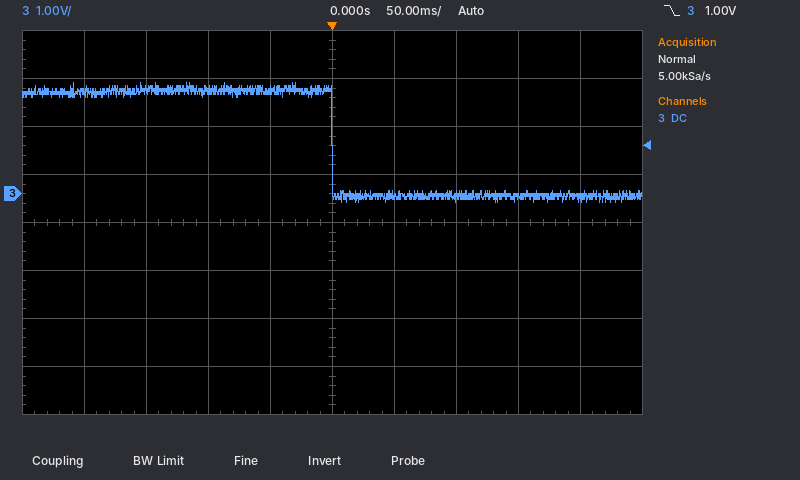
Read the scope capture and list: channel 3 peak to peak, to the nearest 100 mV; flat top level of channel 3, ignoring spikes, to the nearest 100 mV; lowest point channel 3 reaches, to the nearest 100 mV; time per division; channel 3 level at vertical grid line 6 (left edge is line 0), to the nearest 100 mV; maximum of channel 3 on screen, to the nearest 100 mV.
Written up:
2.5 V
2.1 V
-200 mV
50 ms
0.0 V
2.3 V
